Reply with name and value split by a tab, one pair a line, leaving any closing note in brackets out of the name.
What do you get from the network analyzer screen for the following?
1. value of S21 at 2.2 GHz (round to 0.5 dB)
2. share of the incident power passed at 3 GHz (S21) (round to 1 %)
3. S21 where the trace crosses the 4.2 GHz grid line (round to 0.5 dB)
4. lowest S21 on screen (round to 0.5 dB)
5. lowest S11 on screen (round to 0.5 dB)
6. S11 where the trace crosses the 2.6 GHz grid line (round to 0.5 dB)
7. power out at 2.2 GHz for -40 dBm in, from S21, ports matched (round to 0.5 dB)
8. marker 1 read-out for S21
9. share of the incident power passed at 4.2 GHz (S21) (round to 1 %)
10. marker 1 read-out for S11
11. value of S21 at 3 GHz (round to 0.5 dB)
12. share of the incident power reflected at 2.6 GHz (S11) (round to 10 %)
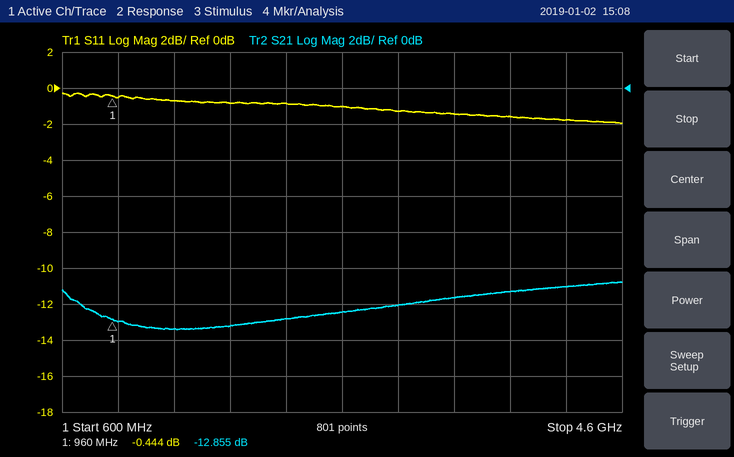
value of S21 at 2.2 GHz	-13.0 dB
share of the incident power passed at 3 GHz (S21)	6 %
S21 where the trace crosses the 4.2 GHz grid line	-11.0 dB
lowest S21 on screen	-13.5 dB
lowest S11 on screen	-2.0 dB
S11 where the trace crosses the 2.6 GHz grid line	-1.0 dB
power out at 2.2 GHz for -40 dBm in, from S21, ports matched	-53.0 dBm
marker 1 read-out for S21	-12.855 dB
share of the incident power passed at 4.2 GHz (S21)	8 %
marker 1 read-out for S11	-0.444 dB
value of S21 at 3 GHz	-12.0 dB
share of the incident power reflected at 2.6 GHz (S11)	80 %
